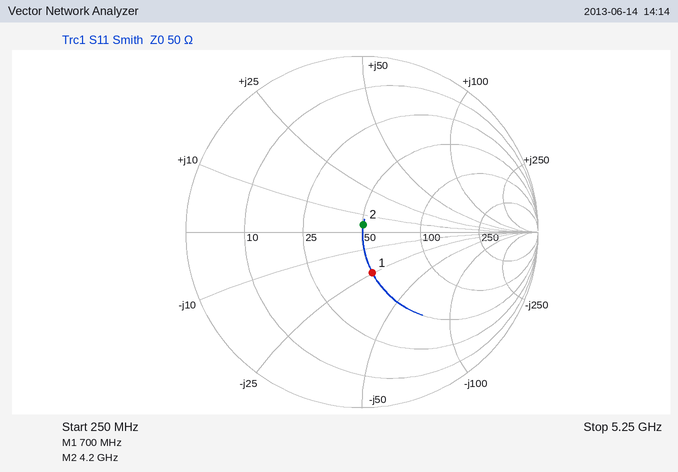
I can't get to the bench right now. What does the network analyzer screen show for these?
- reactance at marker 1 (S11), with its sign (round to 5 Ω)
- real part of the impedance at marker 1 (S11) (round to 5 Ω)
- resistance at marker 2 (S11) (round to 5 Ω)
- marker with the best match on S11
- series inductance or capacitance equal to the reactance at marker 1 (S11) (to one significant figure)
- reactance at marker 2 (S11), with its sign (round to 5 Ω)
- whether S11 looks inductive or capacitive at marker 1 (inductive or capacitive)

-25 Ω
50 Ω
50 Ω
marker 2
9 pF
+5 Ω
capacitive
